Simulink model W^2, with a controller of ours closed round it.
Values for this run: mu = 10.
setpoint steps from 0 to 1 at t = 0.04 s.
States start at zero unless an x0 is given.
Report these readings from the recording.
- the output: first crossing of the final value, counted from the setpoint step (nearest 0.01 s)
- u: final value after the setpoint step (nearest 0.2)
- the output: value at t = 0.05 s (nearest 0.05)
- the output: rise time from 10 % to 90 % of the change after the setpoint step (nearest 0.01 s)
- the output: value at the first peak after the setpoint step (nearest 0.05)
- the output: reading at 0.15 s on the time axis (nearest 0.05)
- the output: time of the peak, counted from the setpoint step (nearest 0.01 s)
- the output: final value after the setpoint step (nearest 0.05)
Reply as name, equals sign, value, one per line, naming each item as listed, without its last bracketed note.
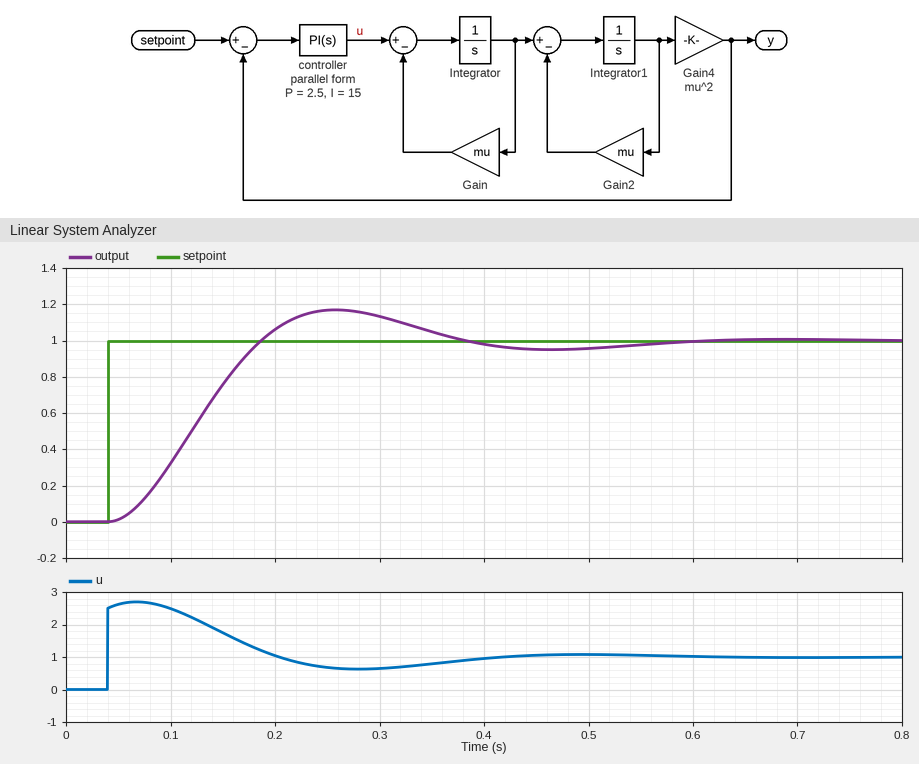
the output: first crossing of the final value, counted from the setpoint step = 0.15 s
u: final value after the setpoint step = 1.0
the output: value at t = 0.05 s = 0.00
the output: rise time from 10 % to 90 % of the change after the setpoint step = 0.10 s
the output: value at the first peak after the setpoint step = 1.15
the output: reading at 0.15 s on the time axis = 0.75
the output: time of the peak, counted from the setpoint step = 0.22 s
the output: final value after the setpoint step = 1.00
